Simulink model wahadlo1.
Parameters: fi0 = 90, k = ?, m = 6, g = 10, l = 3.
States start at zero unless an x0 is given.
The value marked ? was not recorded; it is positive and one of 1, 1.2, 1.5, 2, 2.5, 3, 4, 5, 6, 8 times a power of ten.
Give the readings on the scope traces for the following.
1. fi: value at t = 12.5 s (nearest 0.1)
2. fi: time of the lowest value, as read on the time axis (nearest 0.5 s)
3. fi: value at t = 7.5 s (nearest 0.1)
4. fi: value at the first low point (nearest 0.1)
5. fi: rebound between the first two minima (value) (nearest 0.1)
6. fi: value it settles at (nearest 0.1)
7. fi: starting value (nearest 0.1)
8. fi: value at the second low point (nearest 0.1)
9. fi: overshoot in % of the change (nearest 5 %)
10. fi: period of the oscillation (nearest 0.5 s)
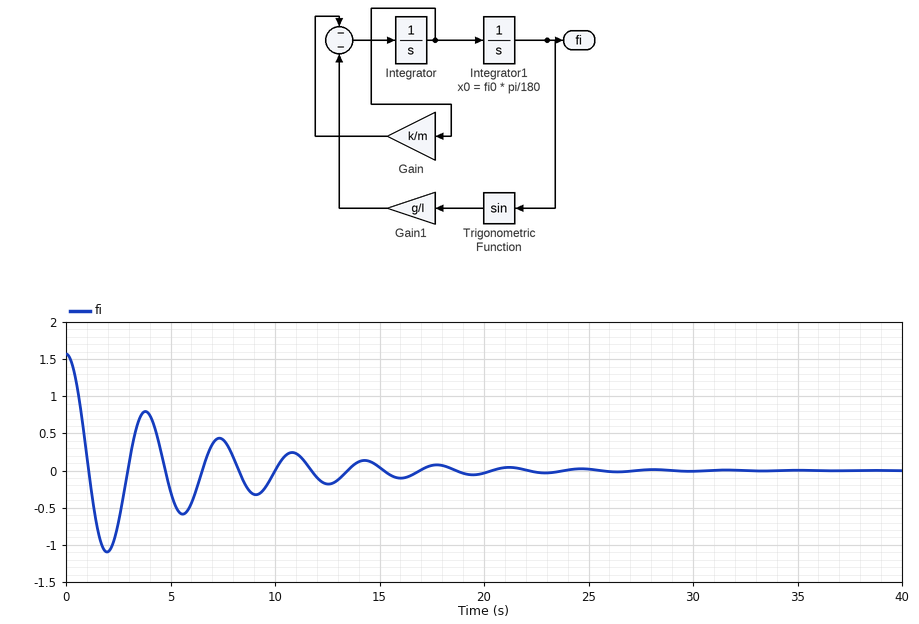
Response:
-0.2
2.0 s
0.4
-1.1
0.8
0.0
1.6
-0.6
70 %
3.5 s
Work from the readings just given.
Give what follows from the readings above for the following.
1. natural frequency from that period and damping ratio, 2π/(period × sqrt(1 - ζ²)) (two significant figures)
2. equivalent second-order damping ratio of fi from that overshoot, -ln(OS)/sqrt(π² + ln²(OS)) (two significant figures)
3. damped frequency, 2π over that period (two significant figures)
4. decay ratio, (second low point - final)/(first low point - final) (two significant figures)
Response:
1.8 rad/s
0.11
1.8 rad/s
0.55
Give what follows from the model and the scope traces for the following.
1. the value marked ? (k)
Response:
2
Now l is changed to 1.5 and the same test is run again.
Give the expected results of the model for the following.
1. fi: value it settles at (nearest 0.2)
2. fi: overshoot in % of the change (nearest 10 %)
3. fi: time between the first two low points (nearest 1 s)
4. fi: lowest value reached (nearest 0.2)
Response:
0.0
80 %
3 s
-1.2
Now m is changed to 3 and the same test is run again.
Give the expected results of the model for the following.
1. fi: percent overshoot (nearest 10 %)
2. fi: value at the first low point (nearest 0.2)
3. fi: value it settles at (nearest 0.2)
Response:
50 %
-0.8
0.0
